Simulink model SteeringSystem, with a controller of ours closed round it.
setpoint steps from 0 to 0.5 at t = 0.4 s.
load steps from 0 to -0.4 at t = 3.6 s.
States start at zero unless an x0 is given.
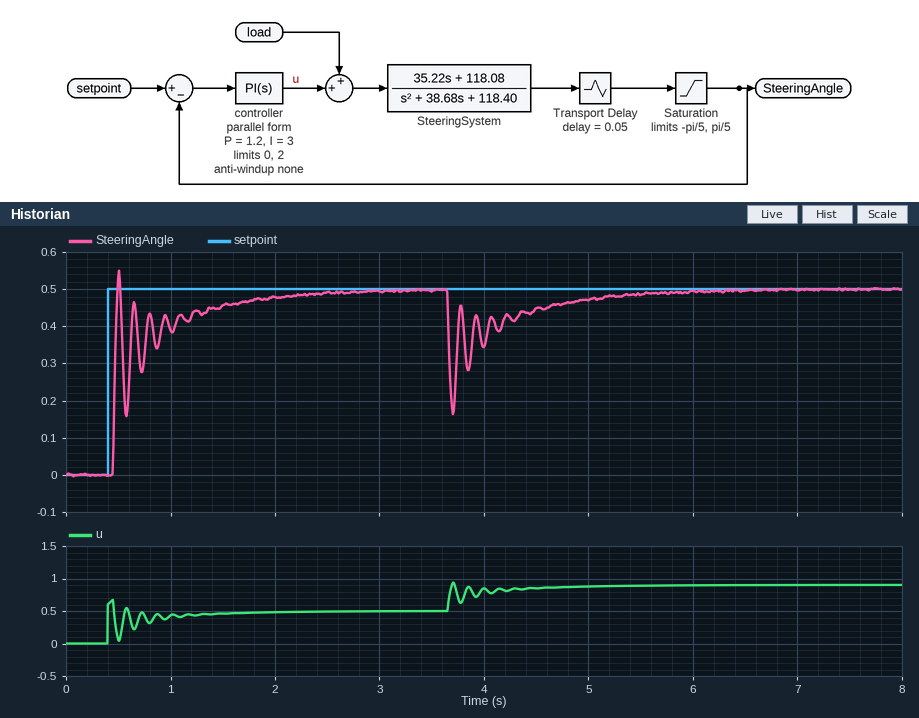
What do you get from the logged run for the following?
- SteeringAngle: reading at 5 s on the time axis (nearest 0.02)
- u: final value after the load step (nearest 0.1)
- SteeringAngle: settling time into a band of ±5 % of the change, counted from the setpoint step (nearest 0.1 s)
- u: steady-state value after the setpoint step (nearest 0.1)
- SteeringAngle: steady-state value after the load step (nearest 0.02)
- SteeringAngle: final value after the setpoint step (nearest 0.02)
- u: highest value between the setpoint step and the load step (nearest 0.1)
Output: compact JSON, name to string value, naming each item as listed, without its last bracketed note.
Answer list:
{"SteeringAngle: reading at 5 s on the time axis": "0.48", "u: final value after the load step": "0.9", "SteeringAngle: settling time into a band of ±5 % of the change, counted from the setpoint step": "1.5 s", "u: steady-state value after the setpoint step": "0.5", "SteeringAngle: steady-state value after the load step": "0.50", "SteeringAngle: final value after the setpoint step": "0.50", "u: highest value between the setpoint step and the load step": "0.7"}
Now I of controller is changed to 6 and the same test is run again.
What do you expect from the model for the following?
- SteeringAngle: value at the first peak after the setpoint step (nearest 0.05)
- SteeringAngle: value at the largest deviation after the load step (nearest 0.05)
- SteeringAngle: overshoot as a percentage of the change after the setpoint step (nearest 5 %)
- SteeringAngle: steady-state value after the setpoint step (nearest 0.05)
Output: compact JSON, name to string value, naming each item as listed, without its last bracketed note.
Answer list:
{"SteeringAngle: value at the first peak after the setpoint step": "0.60", "SteeringAngle: value at the largest deviation after the load step": "0.15", "SteeringAngle: overshoot as a percentage of the change after the setpoint step": "20 %", "SteeringAngle: steady-state value after the setpoint step": "0.50"}
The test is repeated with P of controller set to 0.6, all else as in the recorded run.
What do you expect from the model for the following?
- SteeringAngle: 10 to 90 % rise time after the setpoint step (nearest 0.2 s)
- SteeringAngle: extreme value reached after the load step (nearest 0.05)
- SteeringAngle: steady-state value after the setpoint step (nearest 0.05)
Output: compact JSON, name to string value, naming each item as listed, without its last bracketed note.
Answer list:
{"SteeringAngle: 10 to 90 % rise time after the setpoint step": "0.8 s", "SteeringAngle: extreme value reached after the load step": "0.15", "SteeringAngle: steady-state value after the setpoint step": "0.50"}
